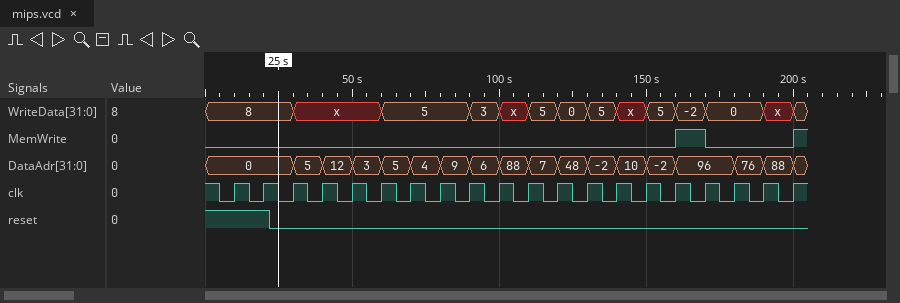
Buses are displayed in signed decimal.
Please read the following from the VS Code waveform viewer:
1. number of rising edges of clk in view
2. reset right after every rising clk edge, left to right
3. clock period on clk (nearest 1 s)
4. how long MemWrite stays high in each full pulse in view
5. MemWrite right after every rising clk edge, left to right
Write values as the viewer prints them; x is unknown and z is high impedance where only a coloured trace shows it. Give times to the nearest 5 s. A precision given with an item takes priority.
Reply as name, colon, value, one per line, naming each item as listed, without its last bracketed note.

number of rising edges of clk in view: 20
reset right after every rising clk edge, left to right: 1 1 0 0 0 0 0 0 0 0 0 0 0 0 0 0 0 0 0 0
clock period on clk: 10 s
how long MemWrite stays high in each full pulse in view: 10 s
MemWrite right after every rising clk edge, left to right: 0 0 0 0 0 0 0 0 0 0 0 0 0 0 0 1 0 0 0 1
